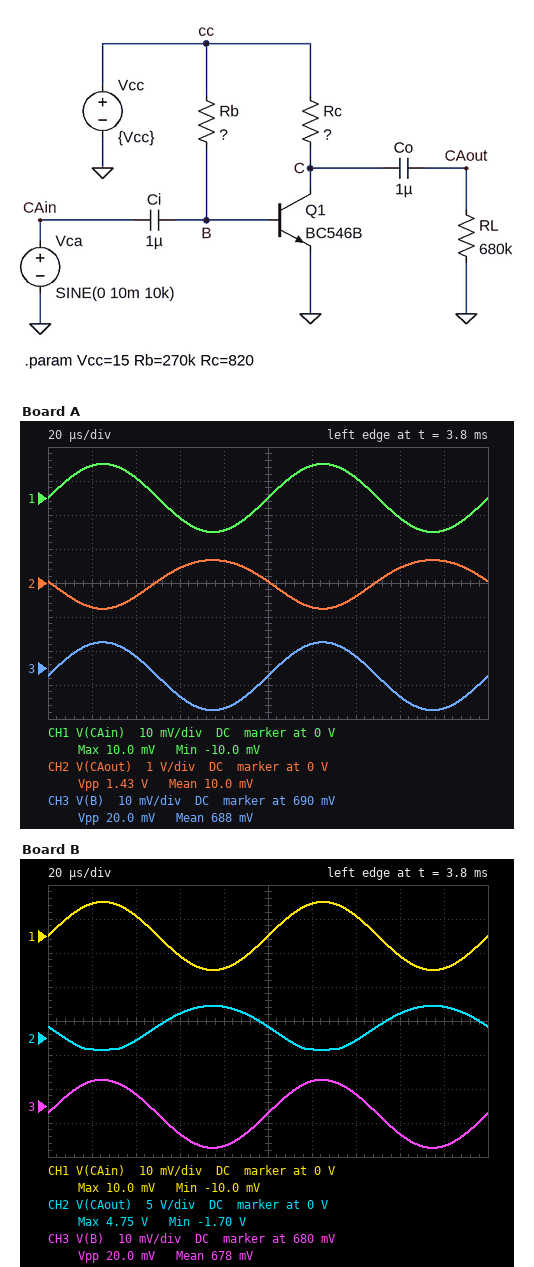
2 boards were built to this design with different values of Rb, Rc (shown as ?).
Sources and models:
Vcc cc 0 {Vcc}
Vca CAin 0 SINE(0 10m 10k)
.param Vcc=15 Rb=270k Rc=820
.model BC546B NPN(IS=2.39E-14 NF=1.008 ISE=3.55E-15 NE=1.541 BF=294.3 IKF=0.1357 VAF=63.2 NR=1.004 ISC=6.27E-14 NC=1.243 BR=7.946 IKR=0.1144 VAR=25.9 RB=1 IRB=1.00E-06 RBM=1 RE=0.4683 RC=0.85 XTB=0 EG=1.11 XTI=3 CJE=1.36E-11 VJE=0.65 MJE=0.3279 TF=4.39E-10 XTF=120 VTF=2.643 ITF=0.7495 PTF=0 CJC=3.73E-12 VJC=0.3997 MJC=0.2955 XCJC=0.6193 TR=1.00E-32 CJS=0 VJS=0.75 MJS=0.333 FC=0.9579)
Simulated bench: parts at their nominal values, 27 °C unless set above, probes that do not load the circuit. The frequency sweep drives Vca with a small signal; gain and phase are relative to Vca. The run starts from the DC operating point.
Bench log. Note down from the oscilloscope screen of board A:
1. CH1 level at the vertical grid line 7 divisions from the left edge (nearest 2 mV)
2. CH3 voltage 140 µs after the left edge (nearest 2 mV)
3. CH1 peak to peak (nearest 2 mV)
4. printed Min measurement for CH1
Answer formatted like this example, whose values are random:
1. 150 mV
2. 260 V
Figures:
1. 6 mV
2. 694 mV
3. 20 mV
4. -10.0 mV
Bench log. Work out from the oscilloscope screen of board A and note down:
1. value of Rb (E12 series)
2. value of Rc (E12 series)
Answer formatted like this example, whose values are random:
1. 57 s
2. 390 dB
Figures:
1. 680 kΩ
2. 330 Ω
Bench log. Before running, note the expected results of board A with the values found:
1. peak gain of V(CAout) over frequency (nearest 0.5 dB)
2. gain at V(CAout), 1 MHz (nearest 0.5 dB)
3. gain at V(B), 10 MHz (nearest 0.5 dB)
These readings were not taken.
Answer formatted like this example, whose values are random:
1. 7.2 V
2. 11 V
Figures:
1. 37.0 dB
2. 37.0 dB
3. 0 dB
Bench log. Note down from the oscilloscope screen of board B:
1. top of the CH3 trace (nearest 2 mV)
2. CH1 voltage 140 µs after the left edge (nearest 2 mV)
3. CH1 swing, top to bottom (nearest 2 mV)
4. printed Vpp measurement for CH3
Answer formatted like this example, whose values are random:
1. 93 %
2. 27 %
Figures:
1. 688 mV
2. 6 mV
3. 20 mV
4. 20.0 mV
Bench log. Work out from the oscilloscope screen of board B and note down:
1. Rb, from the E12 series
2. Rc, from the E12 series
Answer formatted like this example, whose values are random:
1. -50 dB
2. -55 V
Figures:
1. 820 kΩ
2. 2.7 kΩ
